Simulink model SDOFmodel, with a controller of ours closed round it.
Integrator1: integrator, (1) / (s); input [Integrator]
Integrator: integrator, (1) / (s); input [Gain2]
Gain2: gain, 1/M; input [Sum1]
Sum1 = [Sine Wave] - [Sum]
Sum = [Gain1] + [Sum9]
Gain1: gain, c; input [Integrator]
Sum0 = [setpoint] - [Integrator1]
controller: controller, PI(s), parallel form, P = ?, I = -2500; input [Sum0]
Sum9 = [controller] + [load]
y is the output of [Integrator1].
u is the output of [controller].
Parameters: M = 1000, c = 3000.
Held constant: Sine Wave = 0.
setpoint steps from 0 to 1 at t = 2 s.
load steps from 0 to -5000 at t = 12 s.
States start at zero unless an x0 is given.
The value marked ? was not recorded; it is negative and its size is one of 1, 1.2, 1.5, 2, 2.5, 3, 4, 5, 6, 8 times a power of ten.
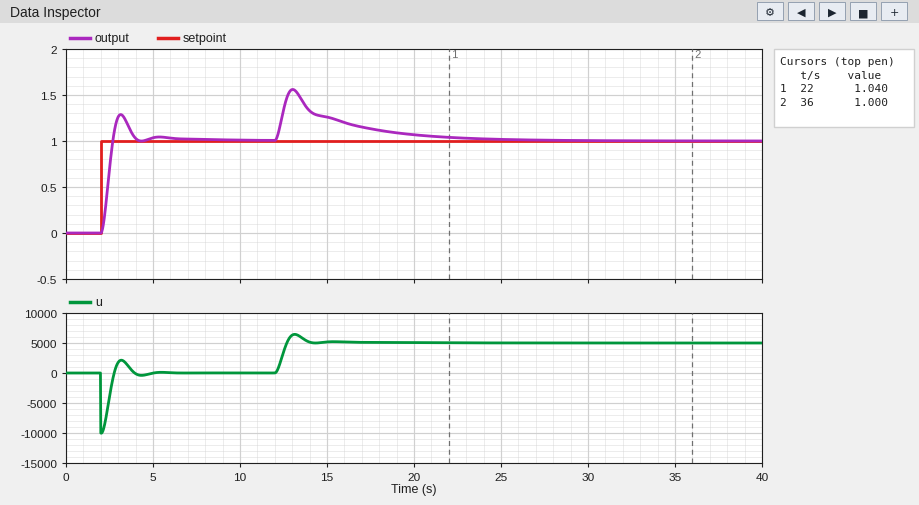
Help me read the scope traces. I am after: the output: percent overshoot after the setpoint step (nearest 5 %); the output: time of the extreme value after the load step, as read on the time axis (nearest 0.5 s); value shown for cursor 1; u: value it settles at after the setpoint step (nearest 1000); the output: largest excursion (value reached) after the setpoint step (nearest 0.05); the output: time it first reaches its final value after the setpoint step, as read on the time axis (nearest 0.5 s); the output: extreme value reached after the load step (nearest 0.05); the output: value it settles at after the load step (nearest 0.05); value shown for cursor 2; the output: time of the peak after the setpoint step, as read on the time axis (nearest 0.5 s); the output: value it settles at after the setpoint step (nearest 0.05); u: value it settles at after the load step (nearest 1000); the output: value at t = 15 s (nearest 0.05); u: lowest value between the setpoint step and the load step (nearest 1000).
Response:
30 %
13.0 s
1.040
0
1.30
2.5 s
1.55
1.00
1.000
3.0 s
1.00
5000
1.25
-10000
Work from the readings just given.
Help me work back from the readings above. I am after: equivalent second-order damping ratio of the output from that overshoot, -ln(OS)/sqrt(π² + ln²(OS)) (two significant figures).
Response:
0.36
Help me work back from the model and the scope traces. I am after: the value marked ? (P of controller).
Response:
-10000
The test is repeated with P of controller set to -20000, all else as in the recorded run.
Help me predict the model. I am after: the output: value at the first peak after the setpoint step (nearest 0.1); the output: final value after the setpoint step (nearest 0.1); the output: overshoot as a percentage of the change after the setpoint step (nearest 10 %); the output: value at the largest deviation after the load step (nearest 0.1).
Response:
1.4
1.0
40 %
1.3
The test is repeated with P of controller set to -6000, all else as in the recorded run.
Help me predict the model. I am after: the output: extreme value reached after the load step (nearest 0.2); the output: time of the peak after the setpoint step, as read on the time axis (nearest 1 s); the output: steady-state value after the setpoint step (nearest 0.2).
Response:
1.8
4 s
1.0
